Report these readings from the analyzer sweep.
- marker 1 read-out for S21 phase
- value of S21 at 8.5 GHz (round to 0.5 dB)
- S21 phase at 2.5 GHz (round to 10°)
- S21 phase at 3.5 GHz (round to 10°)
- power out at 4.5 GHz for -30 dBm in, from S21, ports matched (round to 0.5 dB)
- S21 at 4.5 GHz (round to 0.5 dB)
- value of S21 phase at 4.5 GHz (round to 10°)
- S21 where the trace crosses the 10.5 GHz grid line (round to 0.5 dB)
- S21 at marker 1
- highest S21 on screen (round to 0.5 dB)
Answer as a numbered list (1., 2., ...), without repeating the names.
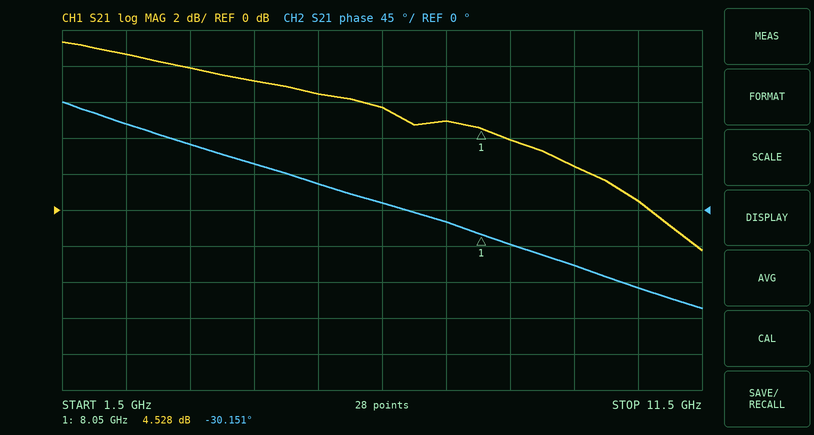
1. -30.151°
2. 4.0 dB
3. 110°
4. 80°
5. -23.0 dBm
6. 7.0 dB
7. 60°
8. 0.5 dB
9. 4.528 dB
10. 9.5 dB
